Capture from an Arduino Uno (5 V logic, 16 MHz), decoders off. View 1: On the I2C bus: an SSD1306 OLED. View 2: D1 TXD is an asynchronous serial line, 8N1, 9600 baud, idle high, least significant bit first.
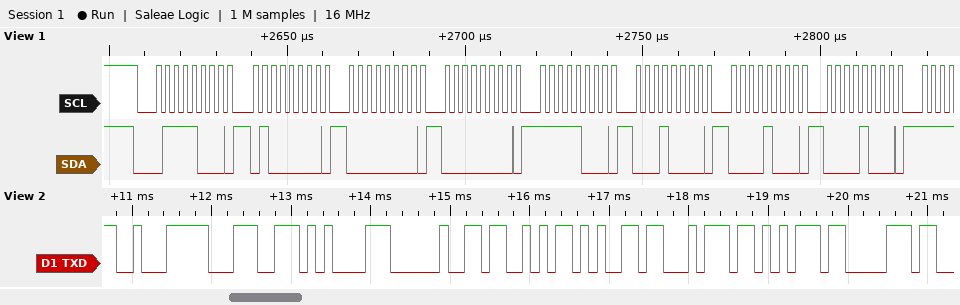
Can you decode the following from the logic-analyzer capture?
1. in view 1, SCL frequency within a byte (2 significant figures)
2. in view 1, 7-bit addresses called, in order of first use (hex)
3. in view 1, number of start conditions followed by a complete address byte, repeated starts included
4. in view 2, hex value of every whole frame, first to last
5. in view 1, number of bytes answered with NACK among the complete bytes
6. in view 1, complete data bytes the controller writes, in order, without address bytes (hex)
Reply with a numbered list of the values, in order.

1. 400 kHz
2. 0x3C
3. 1
4. E2 9C 85 20 53 65 74 75 70
5. 0
6. 40 00 00 F8 10 08 08
